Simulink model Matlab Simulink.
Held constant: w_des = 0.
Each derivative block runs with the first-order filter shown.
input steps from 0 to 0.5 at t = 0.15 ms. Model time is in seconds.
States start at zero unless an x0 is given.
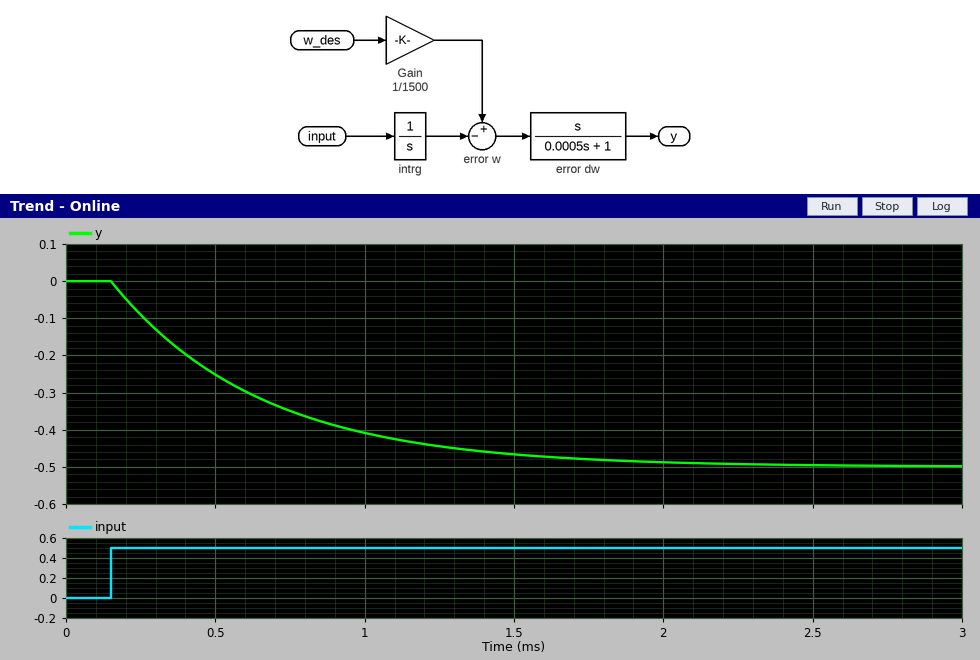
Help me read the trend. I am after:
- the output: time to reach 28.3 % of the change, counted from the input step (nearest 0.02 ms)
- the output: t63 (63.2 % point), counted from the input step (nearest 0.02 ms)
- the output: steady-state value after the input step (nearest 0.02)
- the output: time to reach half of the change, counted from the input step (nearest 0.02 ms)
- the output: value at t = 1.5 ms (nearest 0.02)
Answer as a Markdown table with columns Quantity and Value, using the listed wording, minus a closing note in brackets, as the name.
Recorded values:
| Quantity | Value |
|---|---|
| the output: time to reach 28.3 % of the change, counted from the input step | 0.16 ms |
| the output: t63 (63.2 % point), counted from the input step | 0.50 ms |
| the output: steady-state value after the input step | -0.50 |
| the output: time to reach half of the change, counted from the input step | 0.34 ms |
| the output: value at t = 1.5 ms | -0.46 |
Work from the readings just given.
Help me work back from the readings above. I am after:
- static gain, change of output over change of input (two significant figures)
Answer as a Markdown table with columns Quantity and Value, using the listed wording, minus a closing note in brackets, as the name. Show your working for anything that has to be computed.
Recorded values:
| Quantity | Value |
|---|---|
| static gain, change of output over change of input | (-0.5 - 0) / (0.5 - 0) = -1.0 |
